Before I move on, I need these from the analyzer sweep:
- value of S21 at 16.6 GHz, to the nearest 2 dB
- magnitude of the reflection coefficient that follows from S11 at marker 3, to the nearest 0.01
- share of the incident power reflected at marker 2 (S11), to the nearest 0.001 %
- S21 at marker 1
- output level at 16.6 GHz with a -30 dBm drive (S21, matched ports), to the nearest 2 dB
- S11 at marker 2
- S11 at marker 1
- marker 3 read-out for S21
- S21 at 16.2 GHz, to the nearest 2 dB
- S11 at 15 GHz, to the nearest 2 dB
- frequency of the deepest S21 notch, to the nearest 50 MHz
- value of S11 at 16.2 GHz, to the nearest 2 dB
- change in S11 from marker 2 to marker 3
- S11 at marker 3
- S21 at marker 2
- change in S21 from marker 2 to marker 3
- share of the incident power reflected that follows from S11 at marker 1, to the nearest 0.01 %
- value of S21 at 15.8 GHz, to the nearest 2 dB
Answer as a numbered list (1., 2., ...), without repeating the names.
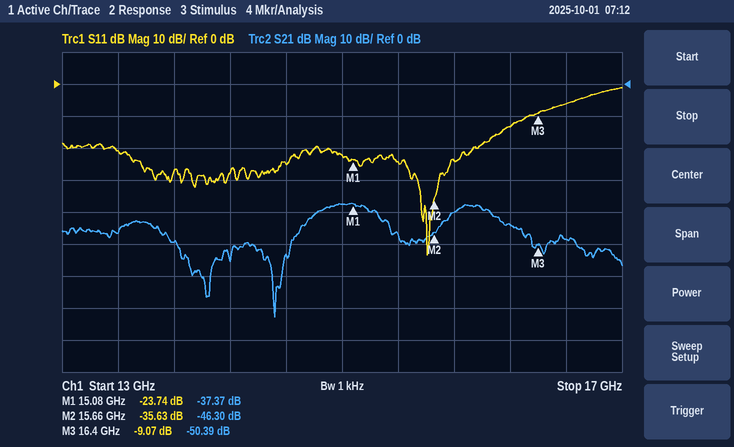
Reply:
1. -48 dB
2. 0.35
3. 0.027 %
4. -37.37 dB
5. -78 dBm
6. -35.63 dB
7. -23.74 dB
8. -50.39 dB
9. -44 dB
10. -22 dB
11. 14.50 GHz
12. -14 dB
13. 26.56 dB
14. -9.07 dB
15. -46.30 dB
16. -4.09 dB
17. 0.42 %
18. -40 dB
